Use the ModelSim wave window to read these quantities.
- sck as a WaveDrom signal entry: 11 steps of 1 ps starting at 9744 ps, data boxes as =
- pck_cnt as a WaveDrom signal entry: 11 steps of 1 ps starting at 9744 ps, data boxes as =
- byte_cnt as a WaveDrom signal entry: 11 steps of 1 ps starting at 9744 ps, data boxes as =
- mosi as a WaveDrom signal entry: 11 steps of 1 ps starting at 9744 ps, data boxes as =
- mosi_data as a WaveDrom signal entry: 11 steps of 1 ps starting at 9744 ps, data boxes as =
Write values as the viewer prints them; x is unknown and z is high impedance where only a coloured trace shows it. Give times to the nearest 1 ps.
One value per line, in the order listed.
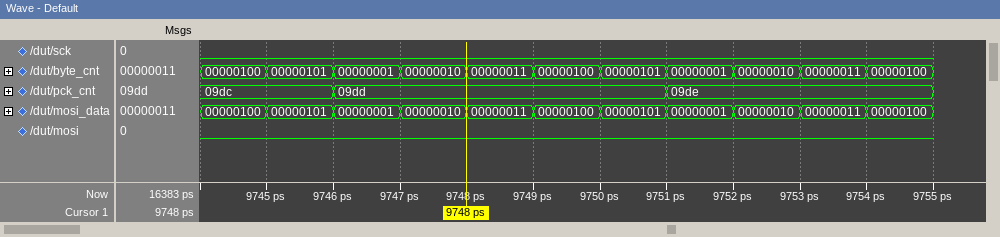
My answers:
{name: 'sck', wave: '0..........'}
{name: 'pck_cnt', wave: '=.=....=...', data: '09dc 09dd 09de'}
{name: 'byte_cnt', wave: '===========', data: '00000100 00000101 00000001 00000010 00000011 00000100 00000101 00000001 00000010 00000011 00000100'}
{name: 'mosi', wave: '0..........'}
{name: 'mosi_data', wave: '===========', data: '00000100 00000101 00000001 00000010 00000011 00000100 00000101 00000001 00000010 00000011 00000100'}
